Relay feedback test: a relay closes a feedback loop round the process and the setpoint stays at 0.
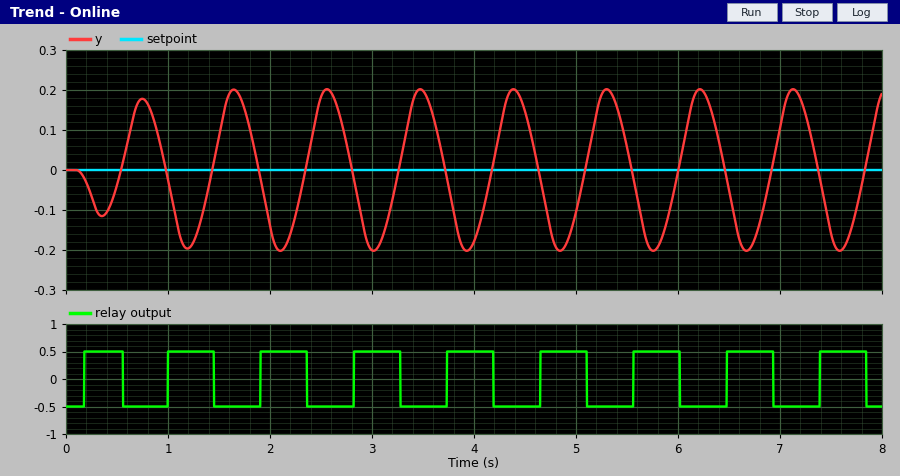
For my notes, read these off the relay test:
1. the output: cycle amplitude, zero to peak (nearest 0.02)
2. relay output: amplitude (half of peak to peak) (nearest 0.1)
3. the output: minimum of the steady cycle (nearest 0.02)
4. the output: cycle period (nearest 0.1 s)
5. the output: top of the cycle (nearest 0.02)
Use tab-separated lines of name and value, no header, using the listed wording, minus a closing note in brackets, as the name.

the output: cycle amplitude, zero to peak	0.20
relay output: amplitude (half of peak to peak)	0.5
the output: minimum of the steady cycle	-0.20
the output: cycle period	0.9 s
the output: top of the cycle	0.20
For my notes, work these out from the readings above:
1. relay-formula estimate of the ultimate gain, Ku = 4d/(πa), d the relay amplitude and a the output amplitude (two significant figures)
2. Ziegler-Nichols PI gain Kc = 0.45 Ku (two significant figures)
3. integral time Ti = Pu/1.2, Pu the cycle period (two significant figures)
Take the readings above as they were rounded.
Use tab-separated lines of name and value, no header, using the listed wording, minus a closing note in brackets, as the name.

relay-formula estimate of the ultimate gain, Ku = 4d/(πa), d the relay amplitude and a the output amplitude	3.2
Ziegler-Nichols PI gain Kc = 0.45 Ku	1.4
integral time Ti = Pu/1.2, Pu the cycle period	0.75 s
